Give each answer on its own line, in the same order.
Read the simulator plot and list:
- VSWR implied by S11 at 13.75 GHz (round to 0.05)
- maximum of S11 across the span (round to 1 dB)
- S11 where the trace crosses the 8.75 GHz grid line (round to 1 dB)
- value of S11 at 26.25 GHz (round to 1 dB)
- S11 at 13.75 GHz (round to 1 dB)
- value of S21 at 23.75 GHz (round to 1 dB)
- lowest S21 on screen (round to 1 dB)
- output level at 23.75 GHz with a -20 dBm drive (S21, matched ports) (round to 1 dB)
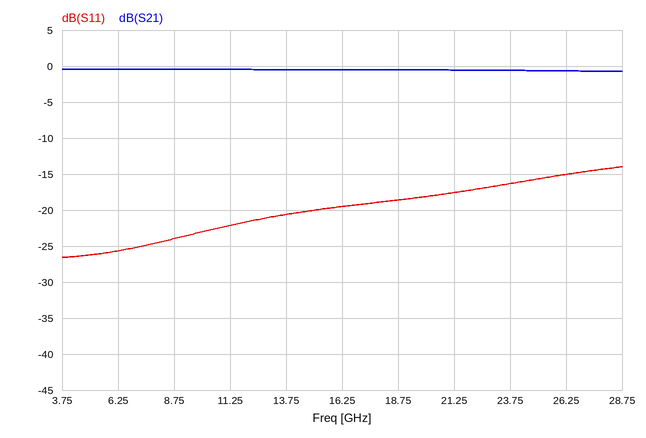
1.20
-14 dB
-24 dB
-15 dB
-21 dB
-1 dB
-1 dB
-21 dBm
